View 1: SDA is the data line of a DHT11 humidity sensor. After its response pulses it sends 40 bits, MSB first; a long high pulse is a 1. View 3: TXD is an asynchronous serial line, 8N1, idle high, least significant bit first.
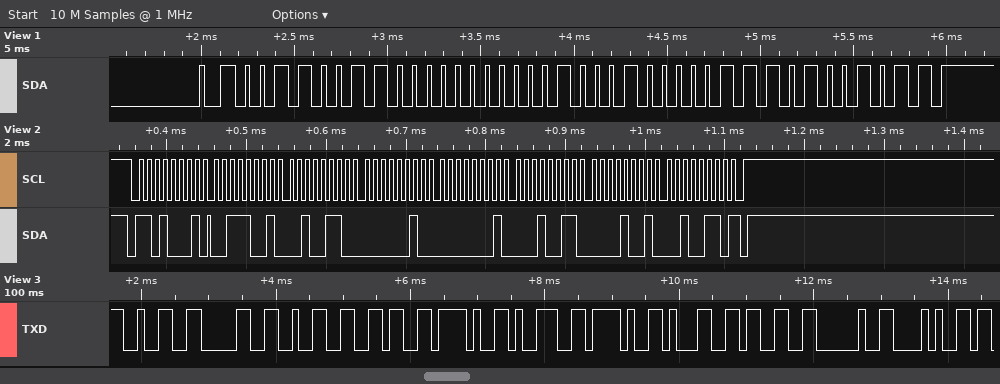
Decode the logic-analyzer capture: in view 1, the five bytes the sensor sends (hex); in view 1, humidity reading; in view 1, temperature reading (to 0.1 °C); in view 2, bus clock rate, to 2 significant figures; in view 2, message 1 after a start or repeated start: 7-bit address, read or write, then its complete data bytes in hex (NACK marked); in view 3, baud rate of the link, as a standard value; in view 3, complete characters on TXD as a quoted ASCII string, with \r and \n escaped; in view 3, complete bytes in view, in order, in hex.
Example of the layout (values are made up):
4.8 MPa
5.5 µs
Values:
33 00 11 07 4B
51 %
17.7 °C
100 kHz
0x68 read: 39 26 02 01 13 09 26 NACK
9600 baud
"2026/9/13 ("
32 30 32 36 2F 39 2F 31 33 20 28
